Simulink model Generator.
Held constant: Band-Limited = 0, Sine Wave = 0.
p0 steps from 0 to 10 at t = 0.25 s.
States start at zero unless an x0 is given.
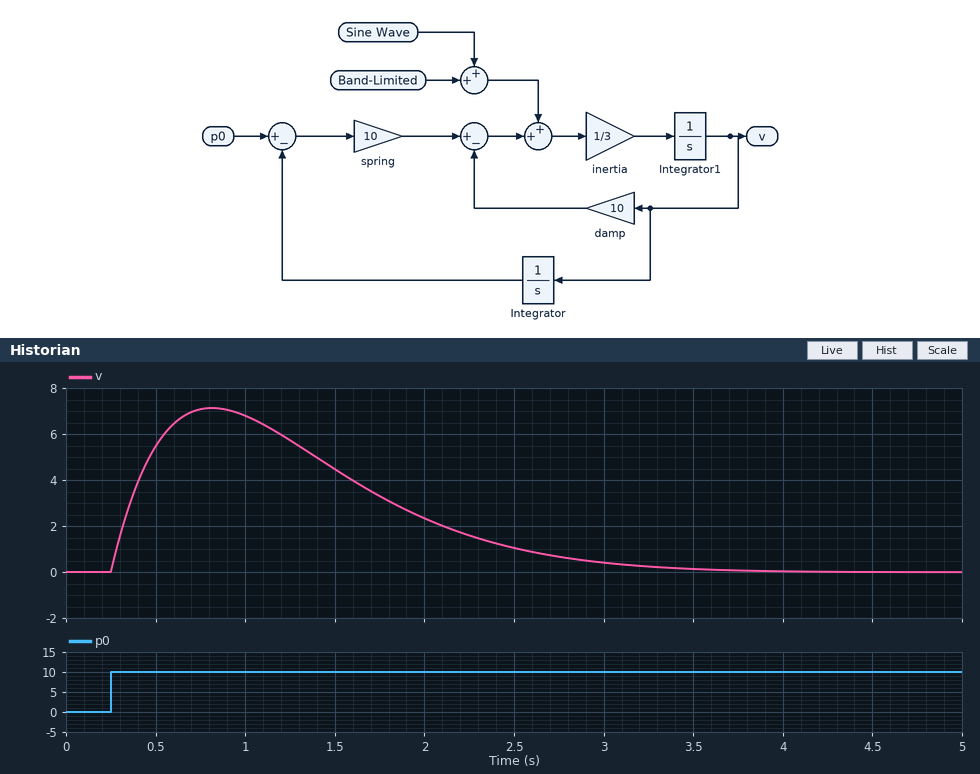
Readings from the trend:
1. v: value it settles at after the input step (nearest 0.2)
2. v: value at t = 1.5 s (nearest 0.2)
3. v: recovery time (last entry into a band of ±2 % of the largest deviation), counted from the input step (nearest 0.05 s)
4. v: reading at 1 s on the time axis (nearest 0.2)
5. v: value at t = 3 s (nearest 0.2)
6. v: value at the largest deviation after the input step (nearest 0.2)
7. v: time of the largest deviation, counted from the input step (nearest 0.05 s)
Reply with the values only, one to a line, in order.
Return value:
0.0
4.4
3.20 s
6.8
0.4
7.2
0.55 s
